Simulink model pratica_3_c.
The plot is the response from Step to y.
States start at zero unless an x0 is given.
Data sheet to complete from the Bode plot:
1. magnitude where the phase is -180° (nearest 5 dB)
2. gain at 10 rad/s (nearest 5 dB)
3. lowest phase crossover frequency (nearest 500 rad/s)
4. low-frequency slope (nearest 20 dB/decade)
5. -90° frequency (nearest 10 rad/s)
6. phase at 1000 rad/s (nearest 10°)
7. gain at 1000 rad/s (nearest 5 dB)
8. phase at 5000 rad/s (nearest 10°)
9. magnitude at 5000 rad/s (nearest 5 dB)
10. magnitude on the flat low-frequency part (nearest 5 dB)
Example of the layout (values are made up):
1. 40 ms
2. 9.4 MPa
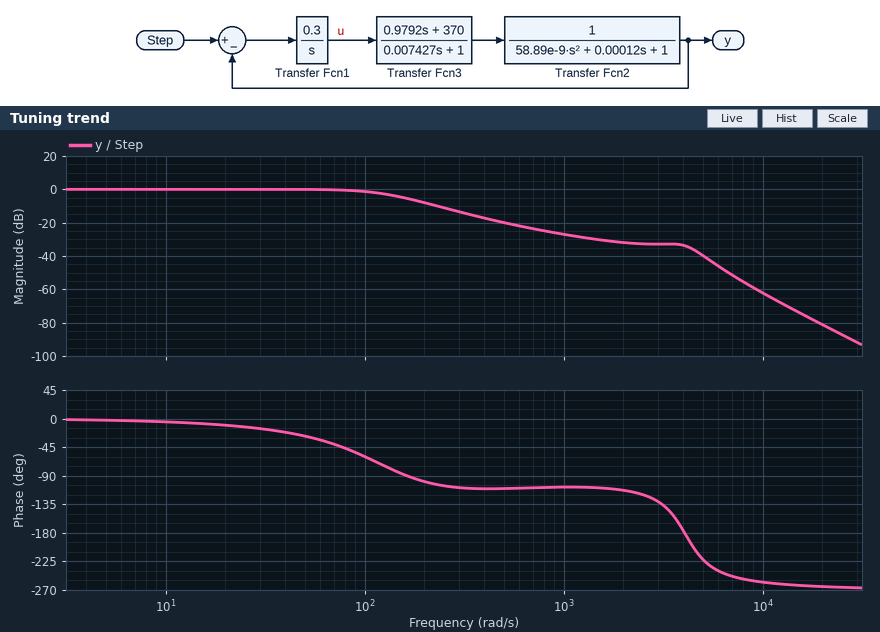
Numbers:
1. -35 dB
2. 0 dB
3. 4000 rad/s
4. 0 dB/decade
5. 160 rad/s
6. -110°
7. -25 dB
8. -220°
9. -40 dB
10. 0 dB
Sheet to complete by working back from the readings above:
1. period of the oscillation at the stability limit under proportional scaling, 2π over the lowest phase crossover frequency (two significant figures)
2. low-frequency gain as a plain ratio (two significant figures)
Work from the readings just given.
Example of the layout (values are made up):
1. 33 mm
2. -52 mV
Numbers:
1. 0.0016 s
2. 1.0
